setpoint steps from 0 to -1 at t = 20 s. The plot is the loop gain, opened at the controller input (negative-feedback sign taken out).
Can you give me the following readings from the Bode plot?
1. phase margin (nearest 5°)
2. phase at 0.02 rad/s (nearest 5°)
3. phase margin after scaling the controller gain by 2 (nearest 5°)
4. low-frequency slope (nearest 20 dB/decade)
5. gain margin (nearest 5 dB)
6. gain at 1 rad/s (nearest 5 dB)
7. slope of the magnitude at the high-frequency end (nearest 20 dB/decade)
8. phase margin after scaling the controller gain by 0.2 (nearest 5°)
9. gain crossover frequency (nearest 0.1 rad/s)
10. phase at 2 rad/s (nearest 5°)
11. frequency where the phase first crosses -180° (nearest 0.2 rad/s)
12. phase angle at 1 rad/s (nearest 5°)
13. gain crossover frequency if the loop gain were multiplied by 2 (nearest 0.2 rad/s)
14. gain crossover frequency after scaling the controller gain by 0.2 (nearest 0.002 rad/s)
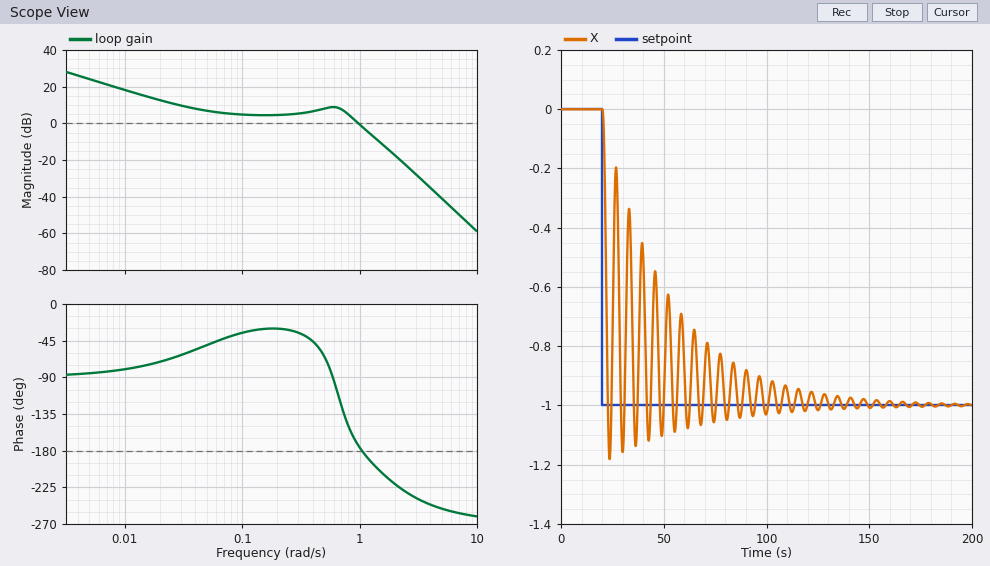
5°
-70°
-15°
-20 dB/decade
0 dB
0 dB
-60 dB/decade
105°
1.0 rad/s
-220°
1.0 rad/s
-175°
1.2 rad/s
0.016 rad/s
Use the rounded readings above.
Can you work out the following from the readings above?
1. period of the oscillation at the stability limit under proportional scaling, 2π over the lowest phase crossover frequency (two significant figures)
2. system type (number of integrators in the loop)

6.3 s
1
